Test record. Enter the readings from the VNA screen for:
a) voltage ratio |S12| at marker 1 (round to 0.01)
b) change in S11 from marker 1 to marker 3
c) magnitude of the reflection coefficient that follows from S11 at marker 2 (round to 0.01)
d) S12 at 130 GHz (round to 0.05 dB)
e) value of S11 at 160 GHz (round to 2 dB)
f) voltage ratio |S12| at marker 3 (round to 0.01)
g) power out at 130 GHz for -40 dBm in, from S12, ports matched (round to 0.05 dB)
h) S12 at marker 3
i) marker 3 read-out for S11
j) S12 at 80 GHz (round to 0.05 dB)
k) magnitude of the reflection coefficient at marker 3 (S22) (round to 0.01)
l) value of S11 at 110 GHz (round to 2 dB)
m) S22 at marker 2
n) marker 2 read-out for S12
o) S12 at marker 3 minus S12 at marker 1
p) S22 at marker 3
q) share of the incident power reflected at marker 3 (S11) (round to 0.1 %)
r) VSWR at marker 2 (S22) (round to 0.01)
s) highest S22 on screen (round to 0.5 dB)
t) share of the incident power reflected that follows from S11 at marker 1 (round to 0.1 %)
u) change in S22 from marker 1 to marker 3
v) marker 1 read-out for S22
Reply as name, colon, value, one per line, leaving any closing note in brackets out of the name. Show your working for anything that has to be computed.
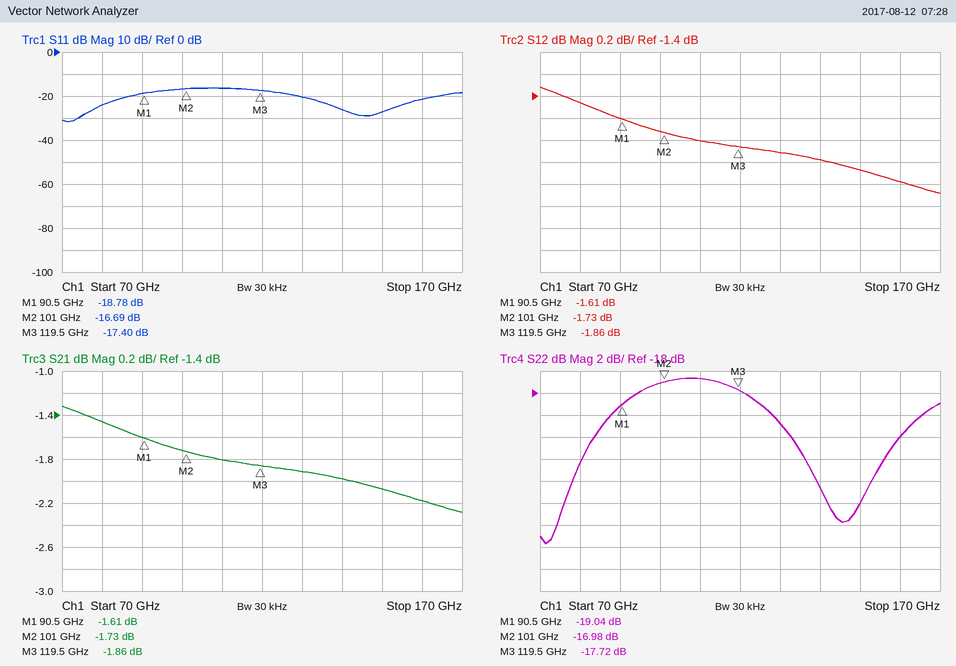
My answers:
voltage ratio |S12| at marker 1: 10^(-1.61/20) ≈ 0.83
change in S11 from marker 1 to marker 3: -17.4 − (-18.78) = 1.38 dB
magnitude of the reflection coefficient that follows from S11 at marker 2: 10^(-16.69/20) ≈ 0.15
S12 at 130 GHz: -1.90 dB
value of S11 at 160 GHz: -22 dB
voltage ratio |S12| at marker 3: 10^(-1.86/20) ≈ 0.81
power out at 130 GHz for -40 dBm in, from S12, ports matched: -40 dBm + (-1.90 dB) = -41.90 dBm
S12 at marker 3: -1.86 dB
marker 3 read-out for S11: -17.40 dB
S12 at 80 GHz: -1.45 dB
magnitude of the reflection coefficient at marker 3 (S22): 10^(-17.72/20) ≈ 0.13
value of S11 at 110 GHz: -16 dB
S22 at marker 2: -16.98 dB
marker 2 read-out for S12: -1.73 dB
S12 at marker 3 minus S12 at marker 1: -1.86 − (-1.61) = -0.25 dB
S22 at marker 3: -17.72 dB
share of the incident power reflected at marker 3 (S11): 10^(-17.4/10) ≈ 1.8 %
VSWR at marker 2 (S22): (1 + 0.1416)/(1 − 0.1416) ≈ 1.33
highest S22 on screen: -16.5 dB
share of the incident power reflected that follows from S11 at marker 1: 10^(-18.78/10) ≈ 1.3 %
change in S22 from marker 1 to marker 3: -17.72 − (-19.04) = 1.32 dB
marker 1 read-out for S22: -19.04 dB
